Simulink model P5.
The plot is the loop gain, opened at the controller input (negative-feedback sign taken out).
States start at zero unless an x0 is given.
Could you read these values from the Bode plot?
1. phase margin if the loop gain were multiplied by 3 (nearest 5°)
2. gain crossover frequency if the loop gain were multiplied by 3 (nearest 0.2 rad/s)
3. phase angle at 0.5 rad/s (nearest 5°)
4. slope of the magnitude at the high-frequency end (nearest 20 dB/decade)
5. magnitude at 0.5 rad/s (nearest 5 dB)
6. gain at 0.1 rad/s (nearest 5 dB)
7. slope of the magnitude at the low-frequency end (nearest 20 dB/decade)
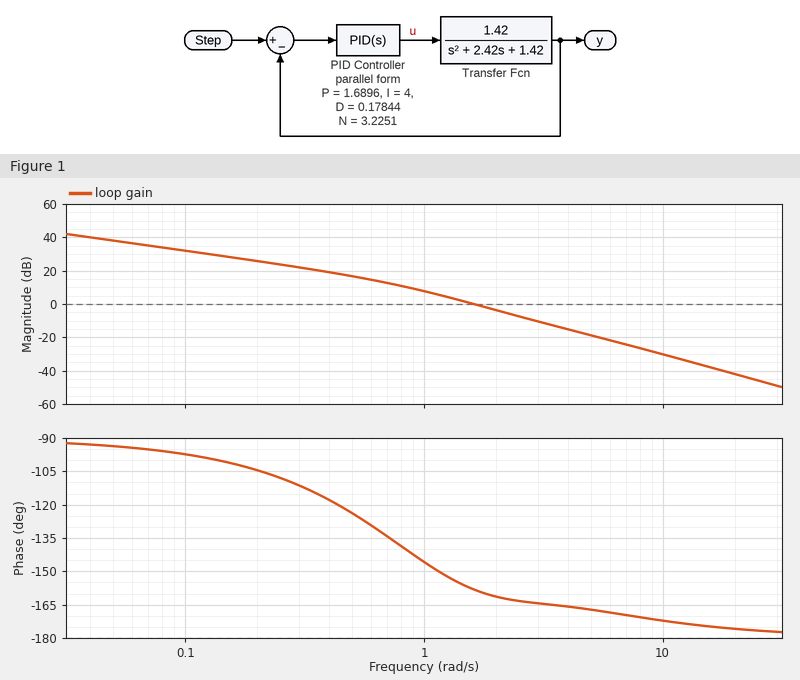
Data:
15°
2.8 rad/s
-125°
-40 dB/decade
15 dB
30 dB
-20 dB/decade
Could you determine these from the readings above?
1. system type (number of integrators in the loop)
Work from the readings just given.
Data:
1
